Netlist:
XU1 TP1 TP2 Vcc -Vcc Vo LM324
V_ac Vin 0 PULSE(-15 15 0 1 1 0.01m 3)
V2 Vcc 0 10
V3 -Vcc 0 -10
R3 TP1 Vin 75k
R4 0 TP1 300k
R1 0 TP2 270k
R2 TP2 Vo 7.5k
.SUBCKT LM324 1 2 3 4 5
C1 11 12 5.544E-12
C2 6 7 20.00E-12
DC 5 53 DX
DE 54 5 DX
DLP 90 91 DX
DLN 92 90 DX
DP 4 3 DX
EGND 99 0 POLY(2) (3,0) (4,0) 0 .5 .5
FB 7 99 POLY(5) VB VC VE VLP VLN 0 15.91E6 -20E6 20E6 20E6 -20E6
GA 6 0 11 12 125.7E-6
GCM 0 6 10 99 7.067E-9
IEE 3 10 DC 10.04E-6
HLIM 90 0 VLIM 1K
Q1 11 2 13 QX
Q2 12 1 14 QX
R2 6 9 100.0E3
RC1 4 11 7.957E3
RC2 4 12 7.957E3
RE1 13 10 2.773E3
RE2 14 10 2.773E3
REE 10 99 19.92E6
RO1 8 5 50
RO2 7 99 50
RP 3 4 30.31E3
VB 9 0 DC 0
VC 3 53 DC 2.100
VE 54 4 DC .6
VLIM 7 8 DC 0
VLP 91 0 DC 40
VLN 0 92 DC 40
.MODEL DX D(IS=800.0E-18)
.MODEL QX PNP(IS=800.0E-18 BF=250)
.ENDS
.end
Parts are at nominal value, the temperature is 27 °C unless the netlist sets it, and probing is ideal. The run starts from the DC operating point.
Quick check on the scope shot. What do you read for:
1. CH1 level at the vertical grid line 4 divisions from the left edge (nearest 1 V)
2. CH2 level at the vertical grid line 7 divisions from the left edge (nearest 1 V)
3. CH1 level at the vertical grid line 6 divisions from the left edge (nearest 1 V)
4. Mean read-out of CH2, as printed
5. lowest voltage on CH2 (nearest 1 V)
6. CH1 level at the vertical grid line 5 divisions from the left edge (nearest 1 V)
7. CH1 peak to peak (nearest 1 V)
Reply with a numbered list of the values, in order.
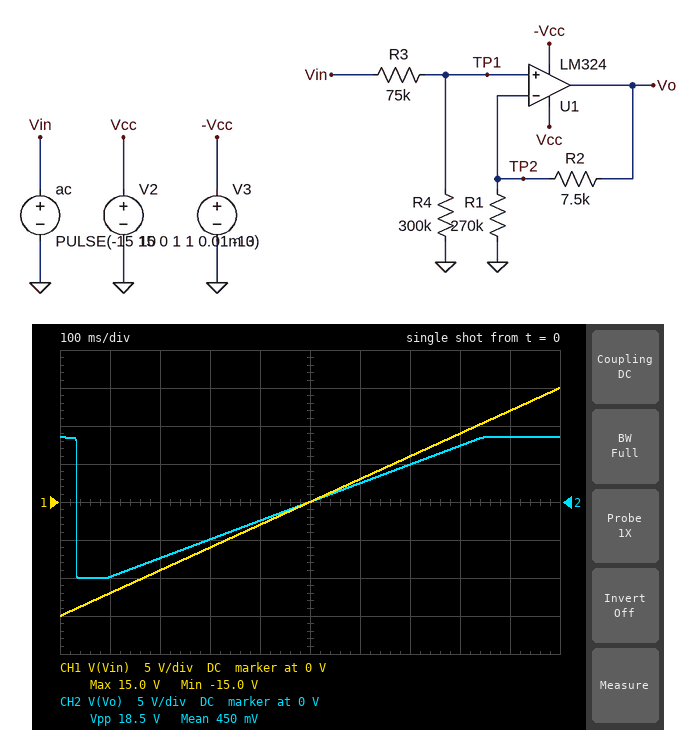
1. -3 V
2. 5 V
3. 3 V
4. 450 mV
5. -10 V
6. 0 V
7. 30 V
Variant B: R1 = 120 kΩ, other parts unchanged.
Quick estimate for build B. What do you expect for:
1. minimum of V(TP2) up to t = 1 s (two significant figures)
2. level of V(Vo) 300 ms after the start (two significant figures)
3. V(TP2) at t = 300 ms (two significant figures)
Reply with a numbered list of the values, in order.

1. -9.4 V
2. -5.1 V
3. -4.8 V
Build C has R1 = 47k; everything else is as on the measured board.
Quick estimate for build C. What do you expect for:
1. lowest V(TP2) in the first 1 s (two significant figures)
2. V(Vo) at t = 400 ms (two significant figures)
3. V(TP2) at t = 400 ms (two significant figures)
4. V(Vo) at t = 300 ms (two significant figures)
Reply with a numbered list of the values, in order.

1. -8.6 V
2. -2.8 V
3. -2.4 V
4. -5.6 V
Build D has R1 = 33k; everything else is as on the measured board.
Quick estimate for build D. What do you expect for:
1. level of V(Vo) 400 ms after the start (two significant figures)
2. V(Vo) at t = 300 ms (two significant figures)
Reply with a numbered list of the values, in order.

1. -2.9 V
2. -5.9 V
